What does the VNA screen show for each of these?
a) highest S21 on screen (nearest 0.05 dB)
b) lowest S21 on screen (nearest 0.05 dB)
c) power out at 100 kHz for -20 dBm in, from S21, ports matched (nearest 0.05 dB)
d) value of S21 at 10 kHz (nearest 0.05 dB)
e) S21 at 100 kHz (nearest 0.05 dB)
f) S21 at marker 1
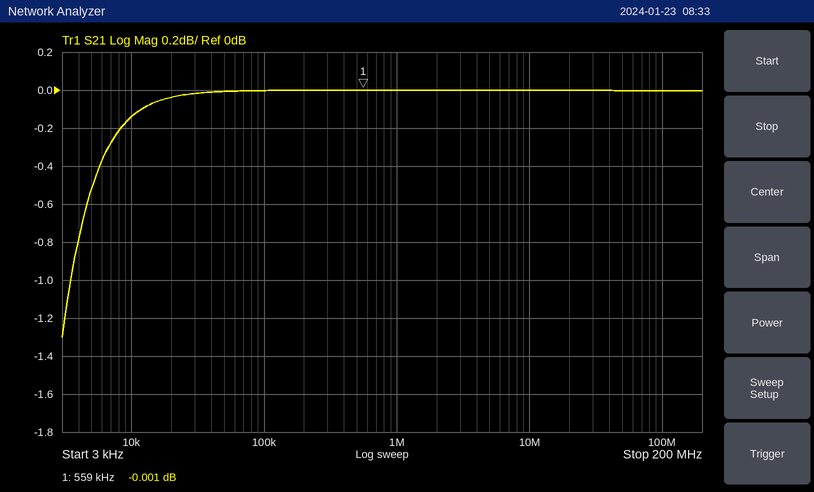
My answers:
0.00 dB
-1.30 dB
-20.00 dBm
-0.15 dB
0.00 dB
-0.001 dB
